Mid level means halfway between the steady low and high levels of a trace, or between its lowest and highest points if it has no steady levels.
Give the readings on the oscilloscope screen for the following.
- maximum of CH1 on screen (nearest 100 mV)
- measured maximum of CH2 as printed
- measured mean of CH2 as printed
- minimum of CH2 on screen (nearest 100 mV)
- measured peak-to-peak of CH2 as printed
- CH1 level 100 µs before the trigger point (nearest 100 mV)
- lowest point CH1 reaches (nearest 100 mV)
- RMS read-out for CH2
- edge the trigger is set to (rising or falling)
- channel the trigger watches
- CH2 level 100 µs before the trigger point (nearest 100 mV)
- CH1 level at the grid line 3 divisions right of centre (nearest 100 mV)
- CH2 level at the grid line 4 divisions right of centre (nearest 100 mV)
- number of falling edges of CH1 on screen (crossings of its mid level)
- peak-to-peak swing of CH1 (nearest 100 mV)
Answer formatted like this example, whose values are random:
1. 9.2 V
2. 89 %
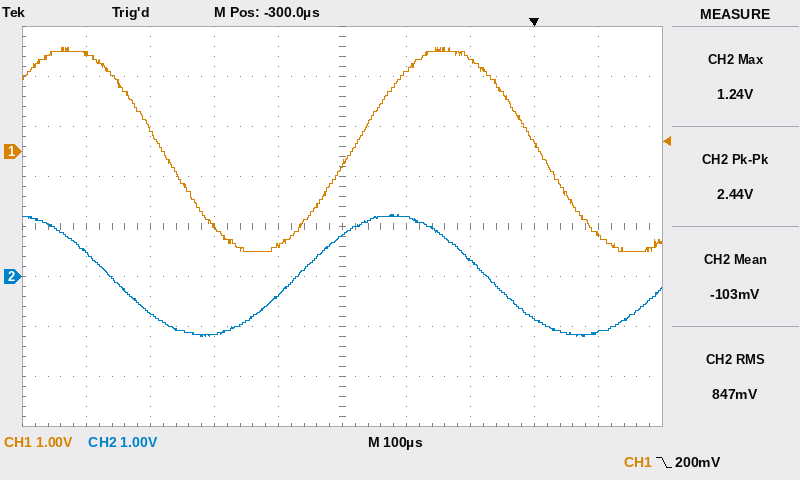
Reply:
1. 2.1 V
2. 1.24 V
3. -103 mV
4. -1.2 V
5. 2.44 V
6. 1.8 V
7. -2.0 V
8. 847 mV
9. falling
10. CH1
11. 300 mV
12. 200 mV
13. -1.1 V
14. 2
15. 4.1 V
